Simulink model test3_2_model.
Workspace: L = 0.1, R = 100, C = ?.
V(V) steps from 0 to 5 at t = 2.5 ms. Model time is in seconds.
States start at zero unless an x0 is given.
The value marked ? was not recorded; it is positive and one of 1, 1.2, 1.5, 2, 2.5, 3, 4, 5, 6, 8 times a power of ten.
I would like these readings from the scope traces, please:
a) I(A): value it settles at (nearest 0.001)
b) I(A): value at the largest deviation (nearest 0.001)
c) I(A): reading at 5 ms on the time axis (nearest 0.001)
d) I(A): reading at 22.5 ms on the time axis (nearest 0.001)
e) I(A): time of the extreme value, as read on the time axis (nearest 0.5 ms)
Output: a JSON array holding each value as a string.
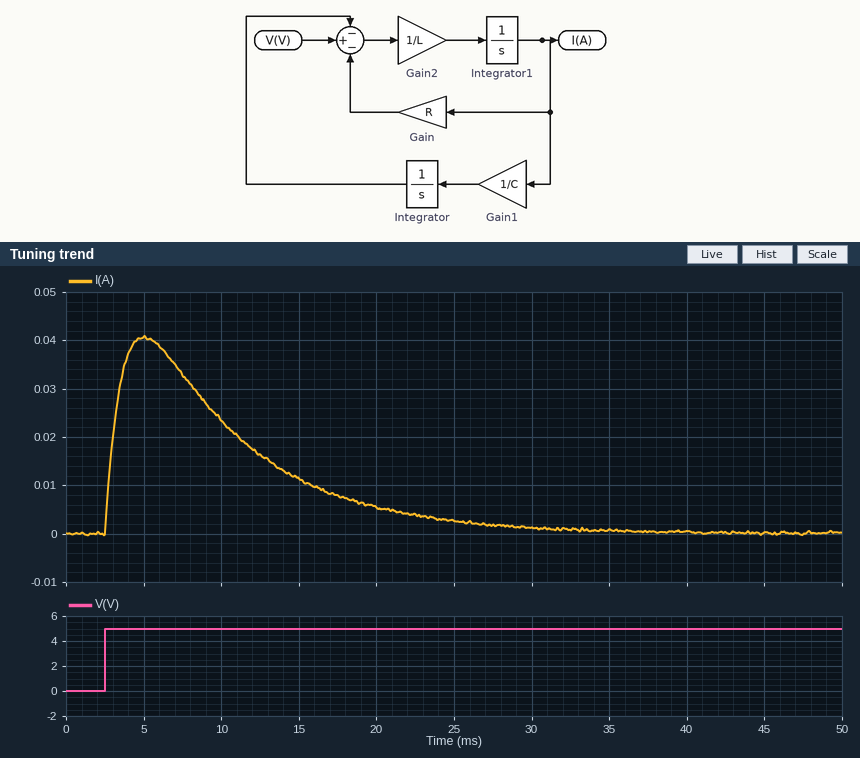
["0.000", "0.041", "0.041", "0.004", "5.0 ms"]
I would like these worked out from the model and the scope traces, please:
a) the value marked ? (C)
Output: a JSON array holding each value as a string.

["8e-05"]
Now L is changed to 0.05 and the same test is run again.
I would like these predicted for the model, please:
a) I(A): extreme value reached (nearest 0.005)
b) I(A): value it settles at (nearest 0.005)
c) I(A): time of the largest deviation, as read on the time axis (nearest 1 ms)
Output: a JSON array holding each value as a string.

["0.045", "0.000", "4 ms"]
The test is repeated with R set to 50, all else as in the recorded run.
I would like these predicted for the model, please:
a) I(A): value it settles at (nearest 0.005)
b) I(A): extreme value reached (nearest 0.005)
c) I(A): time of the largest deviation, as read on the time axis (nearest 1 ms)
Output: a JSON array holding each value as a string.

["0.000", "0.065", "6 ms"]
